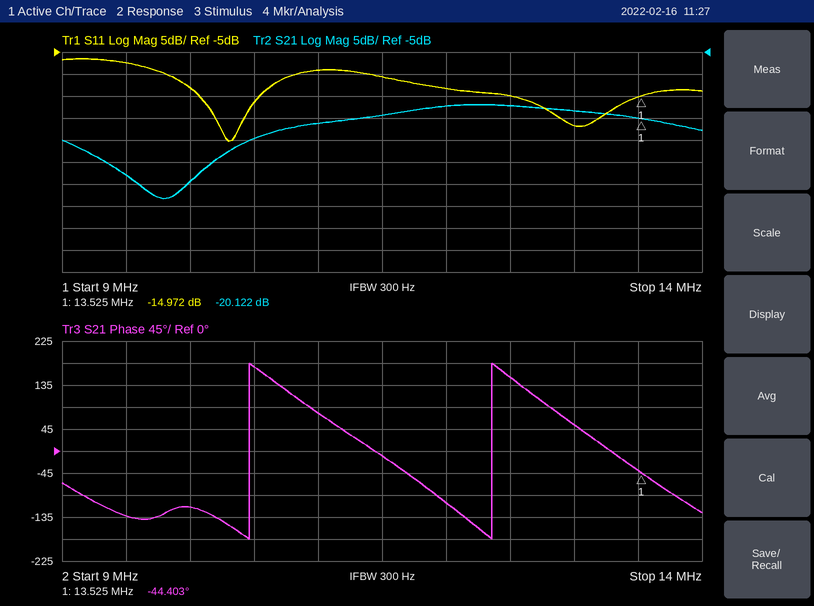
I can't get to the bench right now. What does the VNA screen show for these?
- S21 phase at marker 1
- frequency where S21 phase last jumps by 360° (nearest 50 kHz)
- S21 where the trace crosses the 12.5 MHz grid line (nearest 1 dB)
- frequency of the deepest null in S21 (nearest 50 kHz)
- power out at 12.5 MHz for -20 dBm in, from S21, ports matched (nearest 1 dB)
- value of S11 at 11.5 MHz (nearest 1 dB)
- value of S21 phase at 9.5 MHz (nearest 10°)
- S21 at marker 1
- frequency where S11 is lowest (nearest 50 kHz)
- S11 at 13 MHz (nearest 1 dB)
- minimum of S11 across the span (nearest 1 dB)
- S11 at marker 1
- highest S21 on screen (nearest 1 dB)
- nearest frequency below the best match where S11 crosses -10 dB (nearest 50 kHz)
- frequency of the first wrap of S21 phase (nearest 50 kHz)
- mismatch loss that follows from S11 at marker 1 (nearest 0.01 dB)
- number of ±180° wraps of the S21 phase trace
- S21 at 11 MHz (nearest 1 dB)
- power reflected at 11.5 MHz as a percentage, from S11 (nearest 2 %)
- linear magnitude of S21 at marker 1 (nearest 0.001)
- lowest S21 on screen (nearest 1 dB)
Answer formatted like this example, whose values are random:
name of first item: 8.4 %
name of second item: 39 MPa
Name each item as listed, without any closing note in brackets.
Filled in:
S21 phase at marker 1: -44.403°
frequency where S21 phase last jumps by 360°: 12.35 MHz
S21 where the trace crosses the 12.5 MHz grid line: -17 dB
frequency of the deepest null in S21: 9.80 MHz
power out at 12.5 MHz for -20 dBm in, from S21, ports matched: -37 dBm
value of S11 at 11.5 MHz: -11 dB
value of S21 phase at 9.5 MHz: -130°
S21 at marker 1: -20.122 dB
frequency where S11 is lowest: 10.30 MHz
S11 at 13 MHz: -22 dB
minimum of S11 across the span: -25 dB
S11 at marker 1: -14.972 dB
highest S21 on screen: -17 dB
nearest frequency below the best match where S11 crosses -10 dB: 9.80 MHz
frequency of the first wrap of S21 phase: 10.45 MHz
mismatch loss that follows from S11 at marker 1: 0.14 dB
number of ±180° wraps of the S21 phase trace: 2
S21 at 11 MHz: -21 dB
power reflected at 11.5 MHz as a percentage, from S11: 8 %
linear magnitude of S21 at marker 1: 0.099
lowest S21 on screen: -38 dB
